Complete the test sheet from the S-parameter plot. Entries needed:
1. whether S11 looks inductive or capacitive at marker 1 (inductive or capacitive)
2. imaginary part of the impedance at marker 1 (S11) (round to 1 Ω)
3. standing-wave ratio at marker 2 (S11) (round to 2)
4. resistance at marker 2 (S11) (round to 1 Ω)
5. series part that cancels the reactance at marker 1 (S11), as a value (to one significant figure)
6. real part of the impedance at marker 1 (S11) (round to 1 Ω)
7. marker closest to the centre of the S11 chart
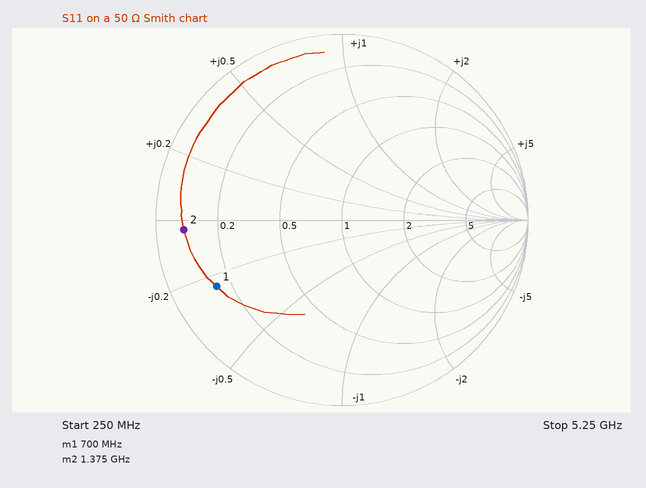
capacitive
-12 Ω
12
4 Ω
3 nH
7 Ω
marker 1
